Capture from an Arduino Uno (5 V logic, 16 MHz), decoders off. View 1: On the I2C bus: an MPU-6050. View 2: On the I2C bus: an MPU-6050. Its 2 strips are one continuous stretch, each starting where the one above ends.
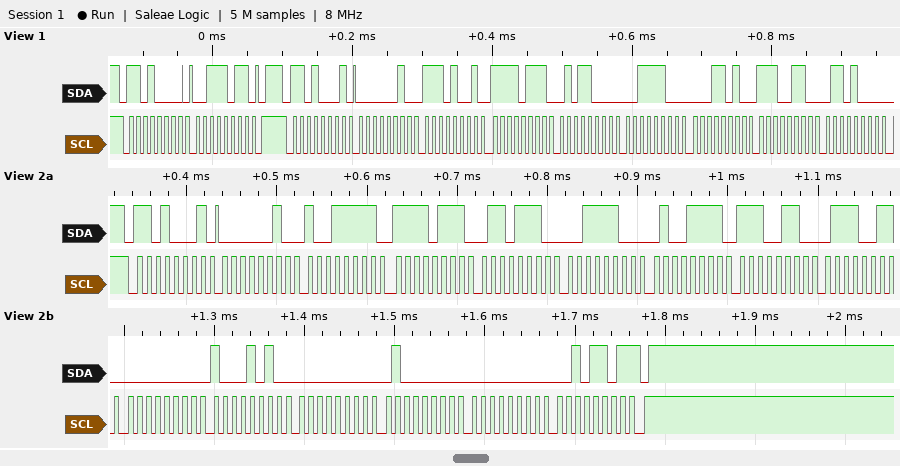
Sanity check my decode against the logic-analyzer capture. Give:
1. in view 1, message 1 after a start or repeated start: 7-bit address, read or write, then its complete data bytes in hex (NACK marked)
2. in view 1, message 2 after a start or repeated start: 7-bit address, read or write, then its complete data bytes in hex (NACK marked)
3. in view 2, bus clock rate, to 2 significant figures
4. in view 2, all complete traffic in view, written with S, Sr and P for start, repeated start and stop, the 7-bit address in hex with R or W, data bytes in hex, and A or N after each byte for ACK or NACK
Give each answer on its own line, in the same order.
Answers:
0x68 write: 3B
0x68 read: 02 E9 F7 58 3C 1A E6 68
100 kHz
S 68R A 02 A 9F A F7 A 6E A 3C A 4F A E6 A 73 A 00 A 8A A 00 A 40 A 00 A 2D N P
